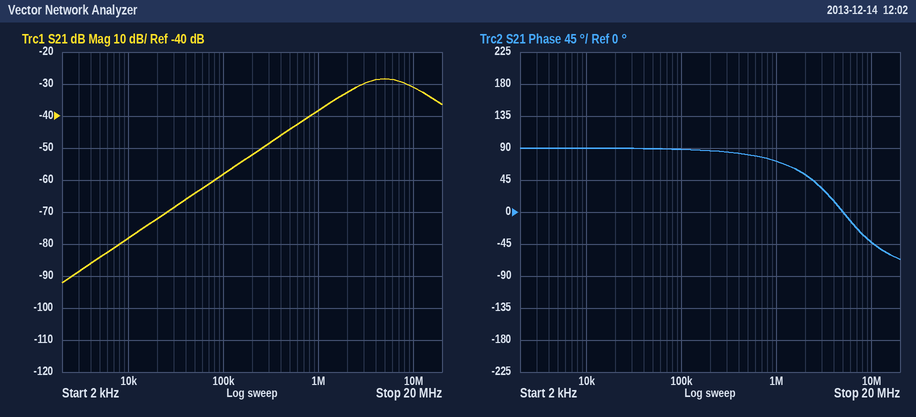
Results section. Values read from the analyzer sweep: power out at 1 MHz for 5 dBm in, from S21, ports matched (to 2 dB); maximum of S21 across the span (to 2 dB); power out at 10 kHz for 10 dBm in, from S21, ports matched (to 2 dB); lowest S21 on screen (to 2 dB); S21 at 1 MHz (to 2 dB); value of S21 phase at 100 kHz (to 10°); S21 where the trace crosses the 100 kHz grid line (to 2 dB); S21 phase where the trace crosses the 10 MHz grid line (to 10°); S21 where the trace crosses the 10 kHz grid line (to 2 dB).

-34 dBm
-28 dB
-68 dBm
-92 dB
-38 dB
90°
-58 dB
-40°
-78 dB
